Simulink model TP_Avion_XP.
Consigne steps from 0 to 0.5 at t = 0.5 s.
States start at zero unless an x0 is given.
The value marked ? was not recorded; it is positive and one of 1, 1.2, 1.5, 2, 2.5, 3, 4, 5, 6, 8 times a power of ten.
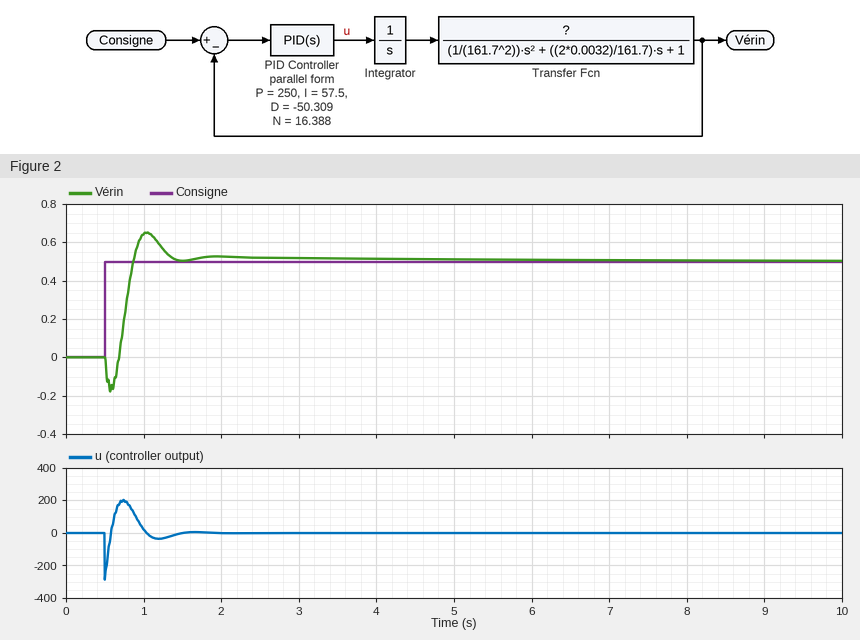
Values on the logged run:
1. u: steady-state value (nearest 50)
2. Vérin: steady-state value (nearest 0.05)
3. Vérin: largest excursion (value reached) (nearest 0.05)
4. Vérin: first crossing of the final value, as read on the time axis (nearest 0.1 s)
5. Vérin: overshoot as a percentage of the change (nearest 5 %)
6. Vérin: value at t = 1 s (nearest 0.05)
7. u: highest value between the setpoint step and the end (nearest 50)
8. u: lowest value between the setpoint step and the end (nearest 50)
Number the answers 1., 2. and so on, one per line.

1. 0
2. 0.50
3. 0.65
4. 0.9 s
5. 30 %
6. 0.65
7. 200
8. -300
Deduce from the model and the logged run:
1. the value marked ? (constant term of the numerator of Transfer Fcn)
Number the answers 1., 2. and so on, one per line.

1. 0.015
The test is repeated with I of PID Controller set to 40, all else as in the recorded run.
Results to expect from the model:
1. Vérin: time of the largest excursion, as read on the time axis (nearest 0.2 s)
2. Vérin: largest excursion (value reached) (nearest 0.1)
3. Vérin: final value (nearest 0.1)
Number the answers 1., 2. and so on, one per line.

1. 1.0 s
2. 0.6
3. 0.5
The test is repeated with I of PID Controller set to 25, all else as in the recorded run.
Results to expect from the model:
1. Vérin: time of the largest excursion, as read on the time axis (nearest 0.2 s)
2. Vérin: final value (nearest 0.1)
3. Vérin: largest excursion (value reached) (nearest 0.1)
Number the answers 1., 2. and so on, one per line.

1. 1.0 s
2. 0.5
3. 0.6
